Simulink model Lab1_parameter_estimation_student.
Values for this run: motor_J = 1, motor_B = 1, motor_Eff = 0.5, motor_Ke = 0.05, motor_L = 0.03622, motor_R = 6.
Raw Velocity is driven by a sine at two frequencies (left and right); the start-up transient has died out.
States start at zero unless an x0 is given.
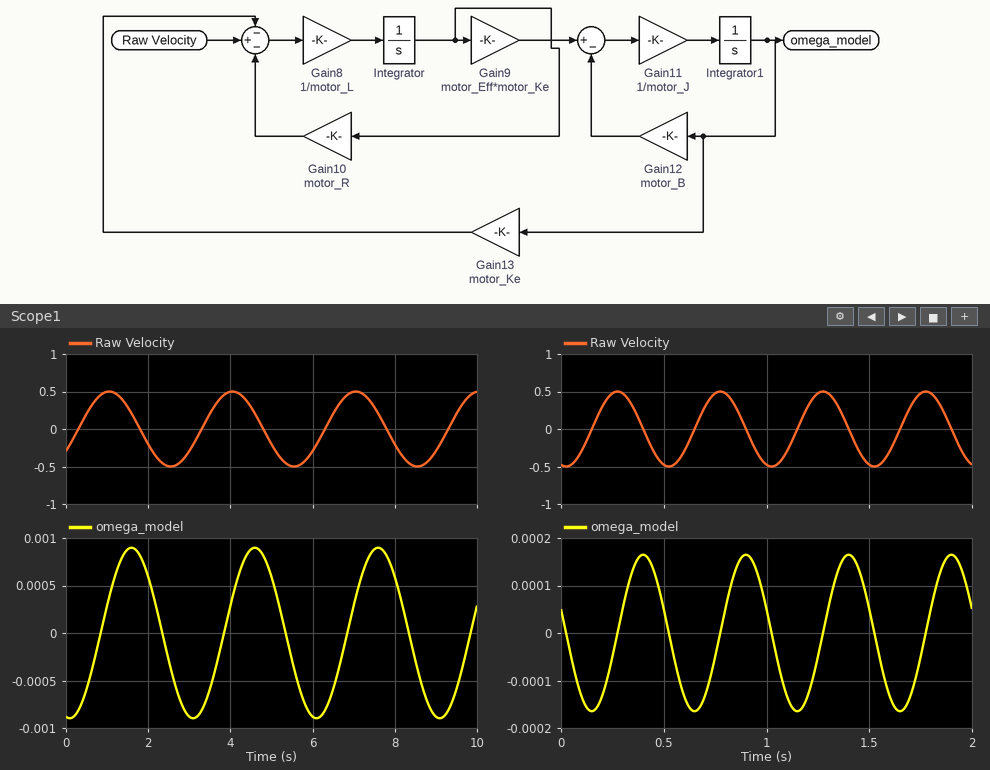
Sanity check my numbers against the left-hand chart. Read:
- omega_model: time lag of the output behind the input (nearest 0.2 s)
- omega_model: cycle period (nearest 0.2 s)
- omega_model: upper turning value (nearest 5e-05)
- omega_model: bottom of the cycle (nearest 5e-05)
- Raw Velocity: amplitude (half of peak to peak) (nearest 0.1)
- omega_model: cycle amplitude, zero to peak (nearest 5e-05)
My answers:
0.6 s
3.0 s
0.00090
-0.00090
0.5
0.00090
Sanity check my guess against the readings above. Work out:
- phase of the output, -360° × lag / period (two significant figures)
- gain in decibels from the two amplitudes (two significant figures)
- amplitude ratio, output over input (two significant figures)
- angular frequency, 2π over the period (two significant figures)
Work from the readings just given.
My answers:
-72°
-55 dB
0.0018
2.1 rad/s
